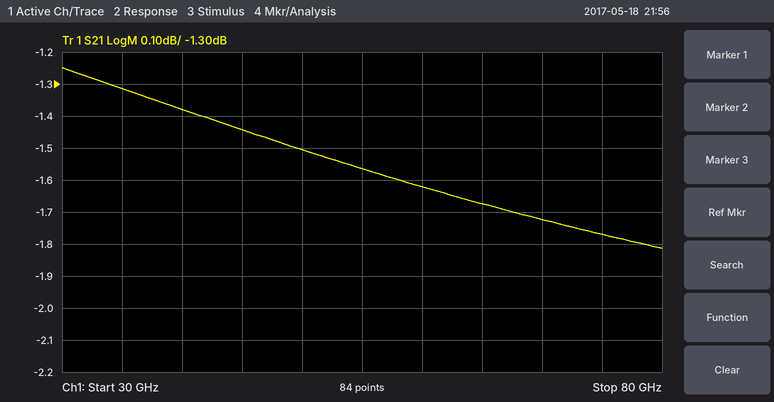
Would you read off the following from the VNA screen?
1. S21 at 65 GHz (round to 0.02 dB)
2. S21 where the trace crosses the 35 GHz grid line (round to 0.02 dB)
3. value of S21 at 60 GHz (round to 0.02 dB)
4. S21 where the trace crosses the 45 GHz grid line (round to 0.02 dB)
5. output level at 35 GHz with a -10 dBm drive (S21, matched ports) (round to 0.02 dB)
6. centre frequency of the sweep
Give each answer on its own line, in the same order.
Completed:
-1.68 dB
-1.32 dB
-1.62 dB
-1.44 dB
-11.32 dBm
55 GHz
